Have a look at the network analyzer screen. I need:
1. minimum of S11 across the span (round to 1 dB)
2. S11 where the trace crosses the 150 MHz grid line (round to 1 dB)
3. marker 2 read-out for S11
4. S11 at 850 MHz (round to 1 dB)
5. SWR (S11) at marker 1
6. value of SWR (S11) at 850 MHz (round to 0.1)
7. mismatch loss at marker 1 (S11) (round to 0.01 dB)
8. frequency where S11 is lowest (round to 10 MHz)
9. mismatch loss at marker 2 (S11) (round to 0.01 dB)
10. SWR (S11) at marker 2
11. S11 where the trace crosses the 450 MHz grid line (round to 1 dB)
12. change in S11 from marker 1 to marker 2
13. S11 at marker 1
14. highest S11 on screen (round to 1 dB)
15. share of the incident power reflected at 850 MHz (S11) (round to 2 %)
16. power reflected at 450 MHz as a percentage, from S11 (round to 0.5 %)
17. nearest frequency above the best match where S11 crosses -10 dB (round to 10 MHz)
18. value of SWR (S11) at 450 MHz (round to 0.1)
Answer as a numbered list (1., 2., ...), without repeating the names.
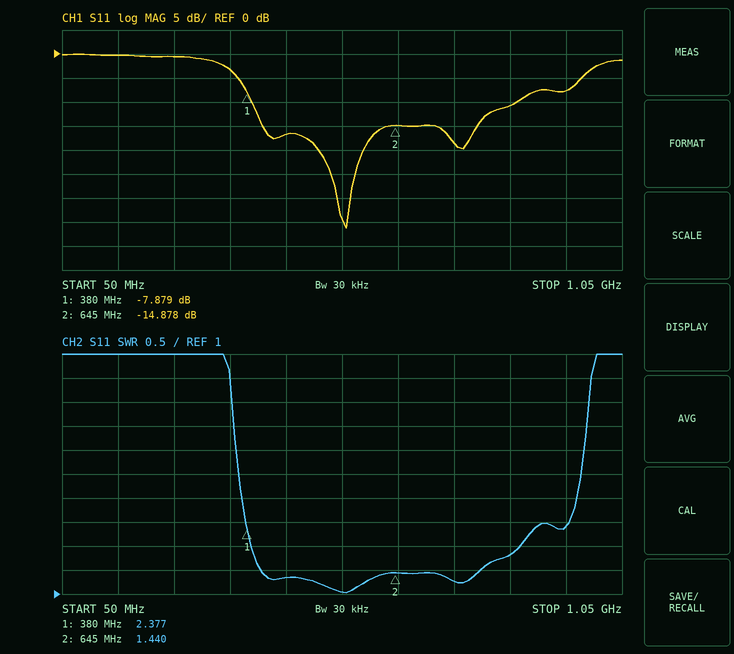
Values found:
1. -36 dB
2. 0 dB
3. -14.878 dB
4. -11 dB
5. 2.377
6. 1.8
7. 0.77 dB
8. 560 MHz
9. 0.14 dB
10. 1.440
11. -17 dB
12. -6.999 dB
13. -7.879 dB
14. 0 dB
15. 8 %
16. 2.0 %
17. 860 MHz
18. 1.3
